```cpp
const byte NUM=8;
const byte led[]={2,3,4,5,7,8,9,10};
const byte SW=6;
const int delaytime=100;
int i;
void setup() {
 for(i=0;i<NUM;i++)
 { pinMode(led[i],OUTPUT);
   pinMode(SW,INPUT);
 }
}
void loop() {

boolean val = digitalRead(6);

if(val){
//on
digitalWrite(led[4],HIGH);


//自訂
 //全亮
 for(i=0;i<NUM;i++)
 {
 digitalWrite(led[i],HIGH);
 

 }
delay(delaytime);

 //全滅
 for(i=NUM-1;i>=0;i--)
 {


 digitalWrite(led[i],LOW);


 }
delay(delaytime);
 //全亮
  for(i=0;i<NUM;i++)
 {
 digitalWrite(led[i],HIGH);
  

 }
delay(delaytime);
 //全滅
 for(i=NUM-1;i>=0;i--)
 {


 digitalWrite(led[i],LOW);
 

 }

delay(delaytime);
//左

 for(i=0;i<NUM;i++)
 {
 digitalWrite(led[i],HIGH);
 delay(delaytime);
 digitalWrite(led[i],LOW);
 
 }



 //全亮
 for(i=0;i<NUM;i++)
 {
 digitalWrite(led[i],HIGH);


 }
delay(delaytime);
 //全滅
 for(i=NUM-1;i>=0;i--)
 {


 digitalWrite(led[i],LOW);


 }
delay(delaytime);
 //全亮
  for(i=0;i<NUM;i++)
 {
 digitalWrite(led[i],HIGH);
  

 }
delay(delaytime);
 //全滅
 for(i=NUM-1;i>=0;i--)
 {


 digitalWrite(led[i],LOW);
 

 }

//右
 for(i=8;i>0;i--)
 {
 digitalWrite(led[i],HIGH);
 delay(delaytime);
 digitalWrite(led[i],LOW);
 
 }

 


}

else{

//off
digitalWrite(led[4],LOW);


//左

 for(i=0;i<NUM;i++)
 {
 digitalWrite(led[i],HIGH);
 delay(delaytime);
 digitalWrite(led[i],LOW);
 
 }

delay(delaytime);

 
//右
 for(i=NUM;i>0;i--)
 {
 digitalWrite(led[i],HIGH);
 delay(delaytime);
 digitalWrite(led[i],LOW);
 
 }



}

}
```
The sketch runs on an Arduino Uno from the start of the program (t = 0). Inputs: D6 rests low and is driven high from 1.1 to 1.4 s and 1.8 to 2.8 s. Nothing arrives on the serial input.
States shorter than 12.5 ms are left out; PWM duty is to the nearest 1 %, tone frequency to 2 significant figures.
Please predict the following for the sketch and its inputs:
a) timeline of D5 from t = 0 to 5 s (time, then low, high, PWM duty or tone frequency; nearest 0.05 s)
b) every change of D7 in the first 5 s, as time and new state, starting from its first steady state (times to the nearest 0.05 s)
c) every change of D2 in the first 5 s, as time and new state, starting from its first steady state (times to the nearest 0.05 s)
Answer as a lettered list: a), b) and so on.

a) 0 s low; 0.3 s high; 0.4 s low; 1.4 s high; 1.5 s low; 2 s high; 2.1 s low; 3.1 s high; 3.2 s low; 3.7 s high; 3.8 s low; 4.8 s high; 4.9 s low
b) 0 s low; 0.4 s high; 0.5 s low; 1.3 s high; 1.4 s low; 2.1 s high; 2.2 s low; 3 s high; 3.1 s low; 3.8 s high; 3.9 s low; 4.7 s high; 4.8 s low
c) 0 s high; 0.1 s low; 1.7 s high; 1.8 s low; 3.4 s high; 3.5 s low
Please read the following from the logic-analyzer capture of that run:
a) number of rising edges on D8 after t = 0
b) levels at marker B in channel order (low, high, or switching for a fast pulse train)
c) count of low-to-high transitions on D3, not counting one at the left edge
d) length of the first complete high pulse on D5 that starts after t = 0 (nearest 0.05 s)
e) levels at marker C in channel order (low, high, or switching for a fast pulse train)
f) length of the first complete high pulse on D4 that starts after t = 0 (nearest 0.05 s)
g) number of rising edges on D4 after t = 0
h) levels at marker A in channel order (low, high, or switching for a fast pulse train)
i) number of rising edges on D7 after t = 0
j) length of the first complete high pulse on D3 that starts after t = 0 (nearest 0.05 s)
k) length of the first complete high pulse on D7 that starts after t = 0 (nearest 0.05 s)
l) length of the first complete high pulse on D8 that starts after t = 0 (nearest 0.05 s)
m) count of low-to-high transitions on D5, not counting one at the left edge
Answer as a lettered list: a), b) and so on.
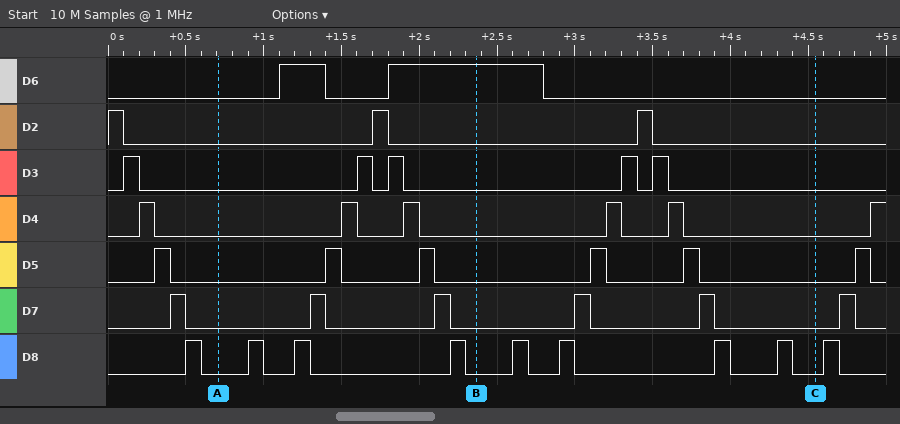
a) 9
b) D6 high, D2 low, D3 low, D4 low, D5 low, D7 low, D8 low
c) 5
d) 0.10 s
e) D6 low, D2 low, D3 low, D4 low, D5 low, D7 low, D8 low
f) 0.10 s
g) 6
h) D6 low, D2 low, D3 low, D4 low, D5 low, D7 low, D8 low
i) 6
j) 0.10 s
k) 0.10 s
l) 0.10 s
m) 6
